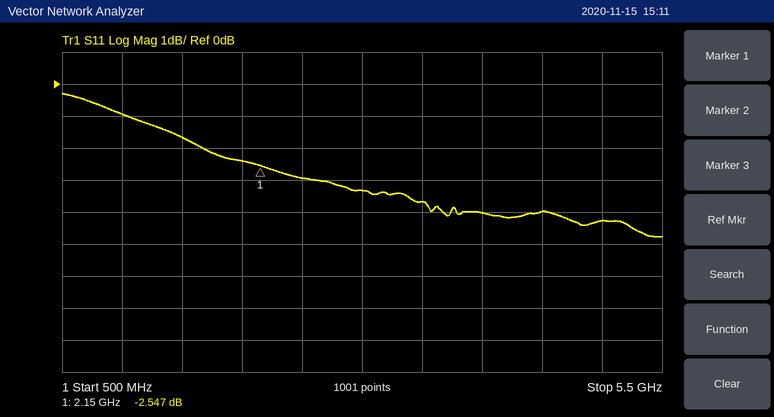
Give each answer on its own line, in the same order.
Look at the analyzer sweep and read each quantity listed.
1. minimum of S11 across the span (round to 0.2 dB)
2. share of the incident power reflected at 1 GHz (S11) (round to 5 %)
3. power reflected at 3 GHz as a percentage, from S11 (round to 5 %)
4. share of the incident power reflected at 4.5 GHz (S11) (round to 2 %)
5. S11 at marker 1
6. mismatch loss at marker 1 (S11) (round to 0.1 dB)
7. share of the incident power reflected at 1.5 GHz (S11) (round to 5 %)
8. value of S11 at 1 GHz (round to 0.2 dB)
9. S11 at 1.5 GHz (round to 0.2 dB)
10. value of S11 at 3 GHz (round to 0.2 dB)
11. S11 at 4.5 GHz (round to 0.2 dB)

-4.8 dB
80 %
45 %
40 %
-2.547 dB
3.5 dB
70 %
-1.0 dB
-1.6 dB
-3.4 dB
-4.0 dB
